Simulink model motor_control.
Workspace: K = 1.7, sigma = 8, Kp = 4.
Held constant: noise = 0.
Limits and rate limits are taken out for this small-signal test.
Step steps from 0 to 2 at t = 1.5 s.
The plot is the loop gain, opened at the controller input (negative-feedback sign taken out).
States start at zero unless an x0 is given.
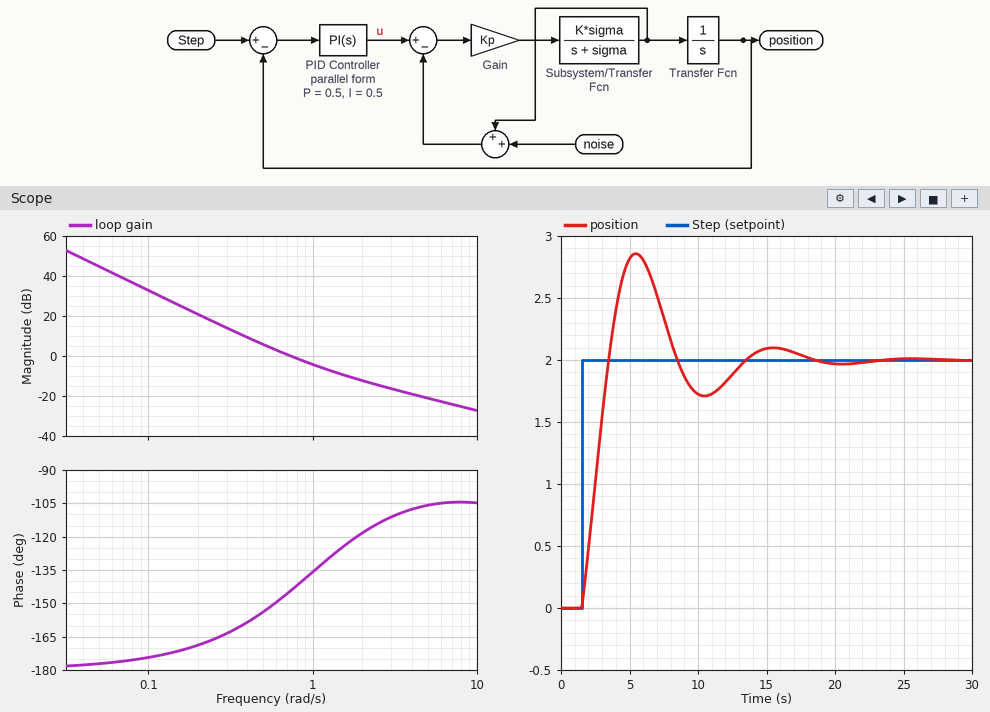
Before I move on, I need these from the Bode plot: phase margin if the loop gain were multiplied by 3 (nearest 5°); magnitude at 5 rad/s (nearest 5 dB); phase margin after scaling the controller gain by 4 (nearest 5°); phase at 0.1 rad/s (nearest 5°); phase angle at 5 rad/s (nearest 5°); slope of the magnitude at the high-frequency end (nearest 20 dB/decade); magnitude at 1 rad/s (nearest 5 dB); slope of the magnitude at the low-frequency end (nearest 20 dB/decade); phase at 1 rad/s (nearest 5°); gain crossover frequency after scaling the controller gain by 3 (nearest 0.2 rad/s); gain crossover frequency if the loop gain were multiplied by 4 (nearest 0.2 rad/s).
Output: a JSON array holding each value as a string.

["55°", "-20 dB", "60°", "-175°", "-105°", "-20 dB/decade", "-5 dB", "-40 dB/decade", "-135°", "1.6 rad/s", "2.0 rad/s"]
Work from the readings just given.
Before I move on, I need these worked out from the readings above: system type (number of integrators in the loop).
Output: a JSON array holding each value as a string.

["2"]
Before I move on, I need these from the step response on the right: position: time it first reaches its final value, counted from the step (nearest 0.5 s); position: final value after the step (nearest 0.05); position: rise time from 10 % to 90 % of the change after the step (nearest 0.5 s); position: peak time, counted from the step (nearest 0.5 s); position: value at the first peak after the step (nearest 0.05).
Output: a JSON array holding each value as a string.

["2.0 s", "2.00", "1.5 s", "4.0 s", "2.85"]
